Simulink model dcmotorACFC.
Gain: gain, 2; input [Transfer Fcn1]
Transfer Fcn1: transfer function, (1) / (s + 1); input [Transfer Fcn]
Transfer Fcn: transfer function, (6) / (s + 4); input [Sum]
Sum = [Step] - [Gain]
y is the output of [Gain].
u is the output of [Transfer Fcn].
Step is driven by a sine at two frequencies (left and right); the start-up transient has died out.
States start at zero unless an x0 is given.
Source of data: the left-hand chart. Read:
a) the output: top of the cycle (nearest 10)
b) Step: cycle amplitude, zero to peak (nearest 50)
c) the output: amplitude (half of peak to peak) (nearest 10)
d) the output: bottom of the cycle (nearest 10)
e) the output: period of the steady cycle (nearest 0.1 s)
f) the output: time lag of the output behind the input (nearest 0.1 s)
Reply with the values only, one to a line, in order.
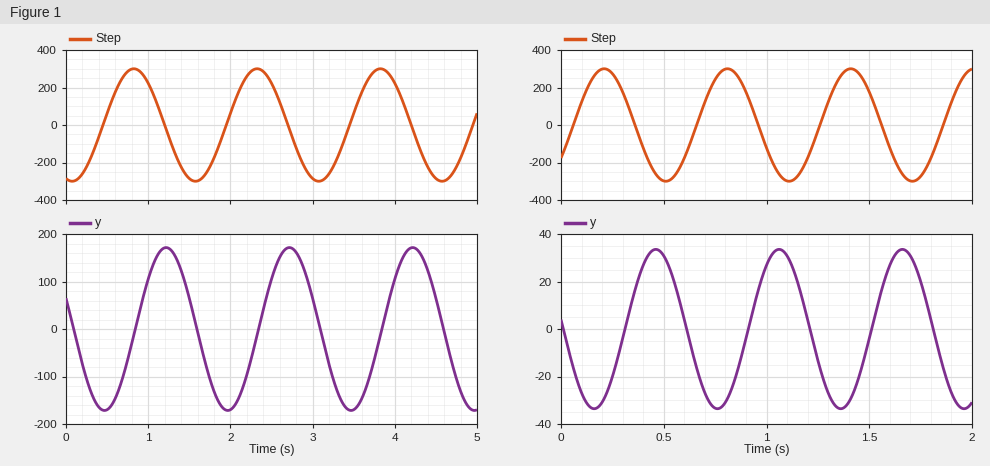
170
300
170
-170
1.5 s
0.4 s
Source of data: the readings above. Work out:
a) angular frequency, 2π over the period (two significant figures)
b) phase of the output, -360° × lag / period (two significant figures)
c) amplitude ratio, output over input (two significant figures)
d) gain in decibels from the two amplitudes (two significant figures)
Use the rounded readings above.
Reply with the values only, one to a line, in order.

4.2 rad/s
-96°
0.57
-4.9 dB
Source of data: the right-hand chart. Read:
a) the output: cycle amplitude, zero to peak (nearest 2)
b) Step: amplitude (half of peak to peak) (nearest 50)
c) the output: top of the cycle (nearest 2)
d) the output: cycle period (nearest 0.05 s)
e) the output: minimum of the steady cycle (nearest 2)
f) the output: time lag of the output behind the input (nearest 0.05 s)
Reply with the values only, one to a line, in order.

34
300
34
0.60 s
-34
0.25 s
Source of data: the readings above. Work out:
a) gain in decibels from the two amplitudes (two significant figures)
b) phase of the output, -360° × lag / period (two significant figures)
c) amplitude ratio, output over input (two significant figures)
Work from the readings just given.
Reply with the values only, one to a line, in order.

-19 dB
-150°
0.11
